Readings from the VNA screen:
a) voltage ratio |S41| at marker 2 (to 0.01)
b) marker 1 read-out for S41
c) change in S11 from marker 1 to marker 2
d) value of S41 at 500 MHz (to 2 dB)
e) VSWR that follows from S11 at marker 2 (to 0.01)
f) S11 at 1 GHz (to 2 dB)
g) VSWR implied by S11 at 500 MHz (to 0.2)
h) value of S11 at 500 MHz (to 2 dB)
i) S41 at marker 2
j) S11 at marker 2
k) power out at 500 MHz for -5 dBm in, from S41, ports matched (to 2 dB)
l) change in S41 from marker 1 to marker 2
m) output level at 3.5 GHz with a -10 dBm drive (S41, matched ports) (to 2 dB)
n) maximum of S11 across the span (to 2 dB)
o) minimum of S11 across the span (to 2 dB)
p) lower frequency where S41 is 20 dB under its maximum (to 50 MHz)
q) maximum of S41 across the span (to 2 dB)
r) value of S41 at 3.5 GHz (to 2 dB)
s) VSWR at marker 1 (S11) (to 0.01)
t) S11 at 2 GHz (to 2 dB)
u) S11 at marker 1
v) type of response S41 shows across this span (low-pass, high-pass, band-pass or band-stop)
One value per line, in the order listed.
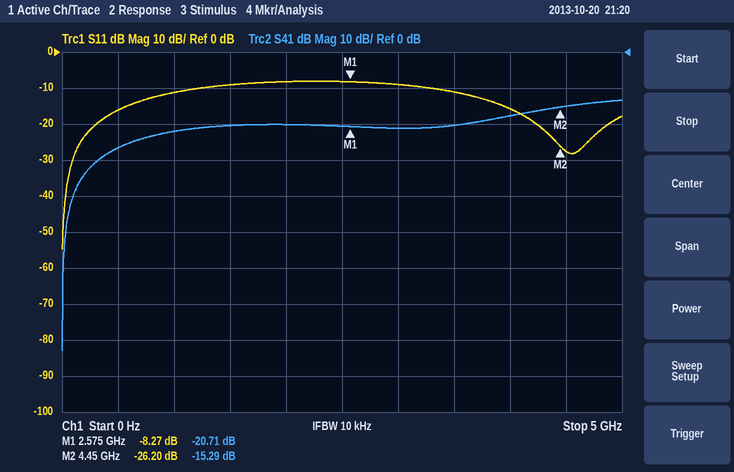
0.17
-20.71 dB
-17.93 dB
-26 dB
1.10
-12 dB
1.4
-16 dB
-15.29 dB
-26.20 dB
-32 dBm
5.42 dB
-30 dBm
-8 dB
-54 dB
200 MHz
-14 dB
-20 dB
2.26
-8 dB
-8.27 dB
high-pass
